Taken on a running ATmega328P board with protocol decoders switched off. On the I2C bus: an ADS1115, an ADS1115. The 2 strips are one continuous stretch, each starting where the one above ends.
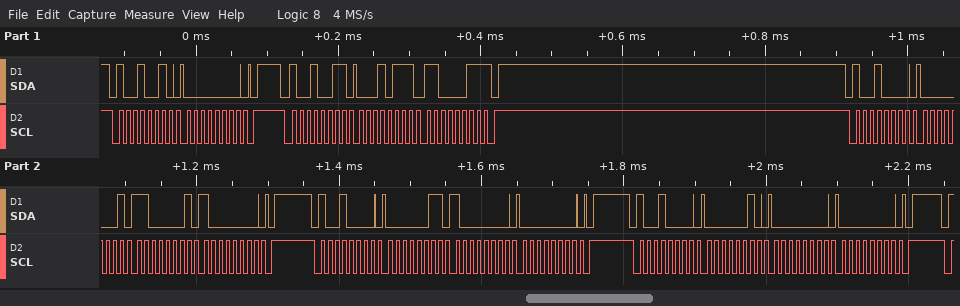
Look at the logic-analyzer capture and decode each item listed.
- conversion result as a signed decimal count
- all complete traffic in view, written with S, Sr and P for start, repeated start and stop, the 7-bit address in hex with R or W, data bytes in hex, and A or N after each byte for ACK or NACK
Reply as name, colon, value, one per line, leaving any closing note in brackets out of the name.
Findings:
conversion result as a signed decimal count: 6083
all complete traffic in view, written with S, Sr and P for start, repeated start and stop, the 7-bit address in hex with R or W, data bytes in hex, and A or N after each byte for ACK or NACK: S 49W A 00 A P S 49R A 17 A C3 N P S 48W A 01 A C1 A 80 A P S 48W A 03 A 80 A 00 A P S 48W A 02 A 00 A 00 A P
